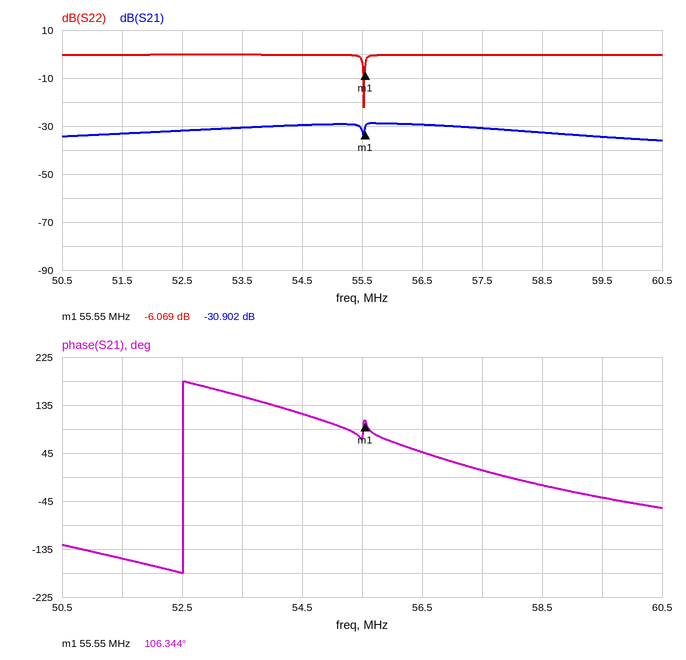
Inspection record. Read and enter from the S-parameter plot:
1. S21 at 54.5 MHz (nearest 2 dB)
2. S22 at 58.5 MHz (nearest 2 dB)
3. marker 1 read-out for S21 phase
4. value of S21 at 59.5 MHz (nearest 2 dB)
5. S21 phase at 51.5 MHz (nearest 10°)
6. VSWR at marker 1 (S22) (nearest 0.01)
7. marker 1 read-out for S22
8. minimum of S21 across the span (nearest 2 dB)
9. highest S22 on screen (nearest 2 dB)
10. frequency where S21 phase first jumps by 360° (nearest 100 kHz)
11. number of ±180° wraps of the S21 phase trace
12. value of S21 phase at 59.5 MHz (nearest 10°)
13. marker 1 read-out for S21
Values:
-30 dB
0 dB
106.344°
-34 dB
-150°
2.98
-6.069 dB
-36 dB
0 dB
52.5 MHz
1
-40°
-30.902 dB
